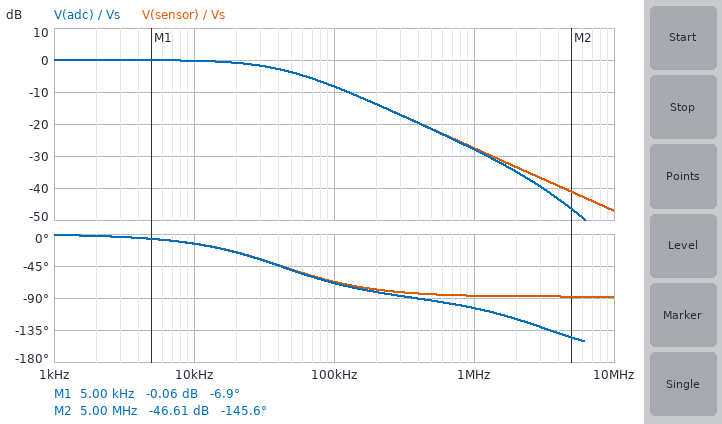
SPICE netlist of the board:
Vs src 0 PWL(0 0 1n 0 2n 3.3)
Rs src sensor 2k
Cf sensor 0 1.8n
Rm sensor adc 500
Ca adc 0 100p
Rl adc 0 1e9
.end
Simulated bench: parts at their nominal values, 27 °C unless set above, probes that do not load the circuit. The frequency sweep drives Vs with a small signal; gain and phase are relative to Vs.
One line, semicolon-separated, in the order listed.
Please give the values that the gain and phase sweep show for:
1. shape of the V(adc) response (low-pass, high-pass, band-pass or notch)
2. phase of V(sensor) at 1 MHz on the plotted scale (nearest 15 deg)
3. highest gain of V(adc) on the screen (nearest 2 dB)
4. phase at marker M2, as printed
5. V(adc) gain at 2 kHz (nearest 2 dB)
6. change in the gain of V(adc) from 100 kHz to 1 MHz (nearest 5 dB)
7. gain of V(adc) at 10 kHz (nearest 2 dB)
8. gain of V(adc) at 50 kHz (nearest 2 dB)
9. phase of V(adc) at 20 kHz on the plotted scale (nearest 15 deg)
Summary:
low-pass; -90 deg; 0 dB; -145.6 deg; 0 dB; -20 dB; 0 dB; -4 dB; -30 deg
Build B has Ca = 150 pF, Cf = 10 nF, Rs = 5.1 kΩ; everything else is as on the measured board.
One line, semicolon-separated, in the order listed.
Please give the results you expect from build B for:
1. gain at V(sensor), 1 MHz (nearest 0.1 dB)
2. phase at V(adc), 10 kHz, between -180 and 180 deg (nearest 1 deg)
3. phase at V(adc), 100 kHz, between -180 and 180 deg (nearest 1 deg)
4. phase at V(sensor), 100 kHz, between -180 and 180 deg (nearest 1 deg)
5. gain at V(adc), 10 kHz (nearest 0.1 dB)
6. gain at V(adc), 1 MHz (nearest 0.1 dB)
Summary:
-50.2 dB; -73 deg; -91 deg; -88 deg; -10.6 dB; -51.1 dB
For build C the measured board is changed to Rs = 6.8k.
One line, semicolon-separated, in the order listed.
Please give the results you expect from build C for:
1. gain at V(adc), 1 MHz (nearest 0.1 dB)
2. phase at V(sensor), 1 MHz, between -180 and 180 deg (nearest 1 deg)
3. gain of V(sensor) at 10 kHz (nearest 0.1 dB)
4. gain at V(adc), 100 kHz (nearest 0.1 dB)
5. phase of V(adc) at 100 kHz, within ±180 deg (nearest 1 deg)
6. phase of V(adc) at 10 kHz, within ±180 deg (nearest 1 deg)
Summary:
-38.6 dB; -88 deg; -2.2 dB; -18.3 dB; -85 deg; -39 deg
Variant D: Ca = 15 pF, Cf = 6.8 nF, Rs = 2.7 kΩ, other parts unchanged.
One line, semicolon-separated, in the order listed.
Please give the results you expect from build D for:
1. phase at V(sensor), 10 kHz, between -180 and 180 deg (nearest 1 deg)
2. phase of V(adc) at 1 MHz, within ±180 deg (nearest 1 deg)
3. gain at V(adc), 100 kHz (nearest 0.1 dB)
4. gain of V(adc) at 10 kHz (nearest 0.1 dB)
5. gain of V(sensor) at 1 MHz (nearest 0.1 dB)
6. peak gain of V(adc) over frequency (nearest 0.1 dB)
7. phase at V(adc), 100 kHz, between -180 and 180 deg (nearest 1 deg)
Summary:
-49 deg; -92 deg; -21.3 dB; -3.7 dB; -41.3 dB; 0 dB; -85 deg
